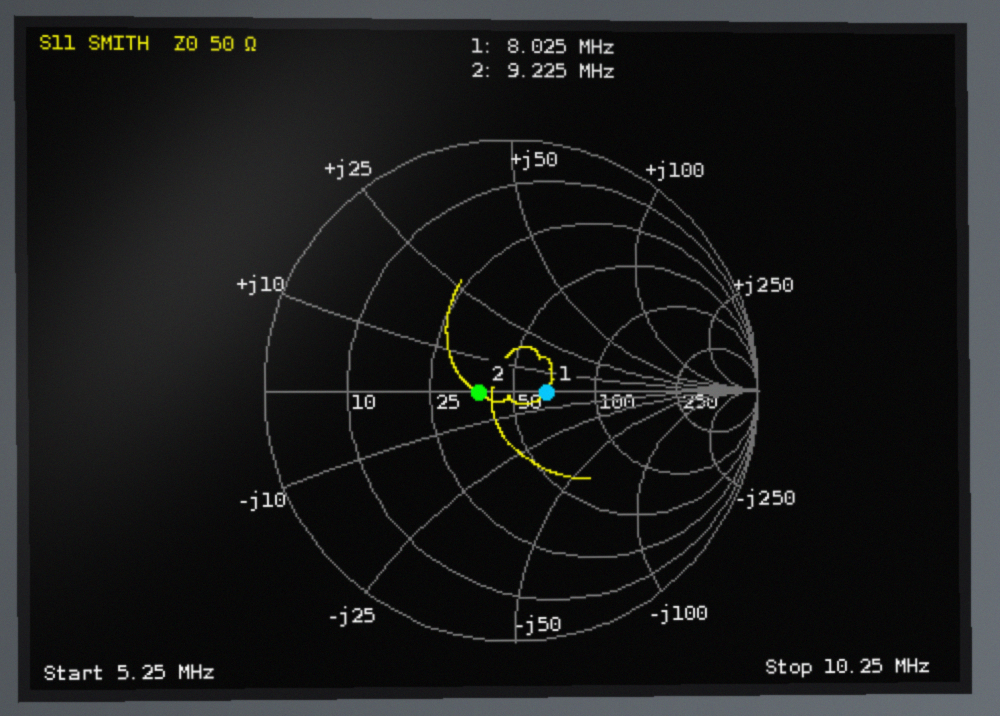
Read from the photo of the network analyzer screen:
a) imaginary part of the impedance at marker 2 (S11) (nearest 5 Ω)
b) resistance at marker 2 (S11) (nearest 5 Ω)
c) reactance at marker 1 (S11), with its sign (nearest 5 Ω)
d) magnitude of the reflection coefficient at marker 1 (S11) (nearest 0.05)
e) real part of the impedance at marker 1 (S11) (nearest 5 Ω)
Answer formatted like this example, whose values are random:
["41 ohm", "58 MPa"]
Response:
["0 Ω", "40 Ω", "0 Ω", "0.15", "65 Ω"]
